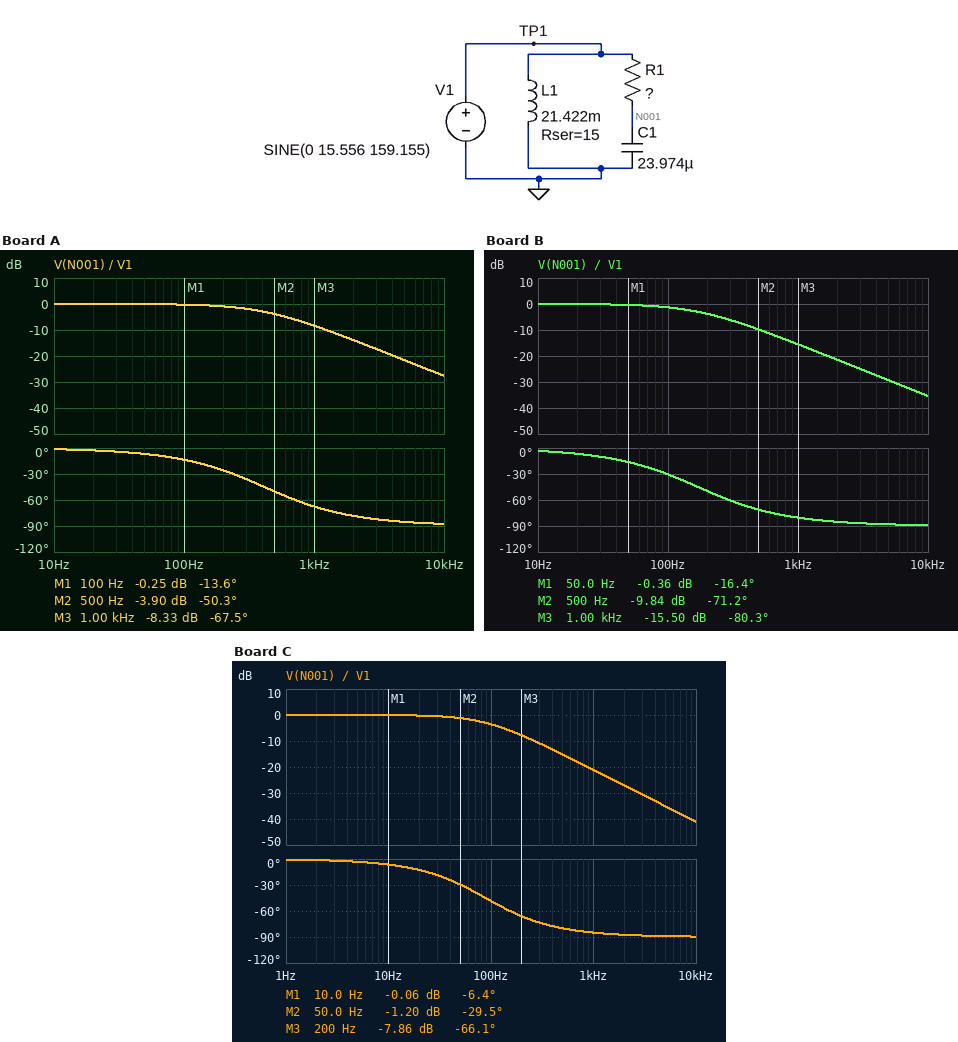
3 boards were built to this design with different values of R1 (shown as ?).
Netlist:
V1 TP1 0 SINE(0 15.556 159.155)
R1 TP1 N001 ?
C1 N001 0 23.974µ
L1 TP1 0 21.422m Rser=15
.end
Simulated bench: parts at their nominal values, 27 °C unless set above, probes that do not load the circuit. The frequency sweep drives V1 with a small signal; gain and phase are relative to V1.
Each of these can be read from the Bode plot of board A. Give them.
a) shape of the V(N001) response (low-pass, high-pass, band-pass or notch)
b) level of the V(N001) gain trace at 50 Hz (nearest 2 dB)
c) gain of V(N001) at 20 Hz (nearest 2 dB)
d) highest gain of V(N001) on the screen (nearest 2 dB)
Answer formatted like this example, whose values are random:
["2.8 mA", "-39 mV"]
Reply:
["low-pass", "0 dB", "0 dB", "0 dB"]
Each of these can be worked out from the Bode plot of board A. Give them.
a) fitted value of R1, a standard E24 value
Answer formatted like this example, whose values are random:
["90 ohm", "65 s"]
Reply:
["16 Ω"]
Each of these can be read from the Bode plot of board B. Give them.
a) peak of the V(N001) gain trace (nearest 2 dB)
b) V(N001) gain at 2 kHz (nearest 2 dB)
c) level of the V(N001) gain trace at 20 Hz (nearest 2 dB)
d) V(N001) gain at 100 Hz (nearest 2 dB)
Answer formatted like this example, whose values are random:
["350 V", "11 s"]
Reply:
["0 dB", "-22 dB", "0 dB", "-2 dB"]
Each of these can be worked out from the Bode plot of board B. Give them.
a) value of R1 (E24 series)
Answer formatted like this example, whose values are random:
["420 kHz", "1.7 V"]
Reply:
["39 Ω"]
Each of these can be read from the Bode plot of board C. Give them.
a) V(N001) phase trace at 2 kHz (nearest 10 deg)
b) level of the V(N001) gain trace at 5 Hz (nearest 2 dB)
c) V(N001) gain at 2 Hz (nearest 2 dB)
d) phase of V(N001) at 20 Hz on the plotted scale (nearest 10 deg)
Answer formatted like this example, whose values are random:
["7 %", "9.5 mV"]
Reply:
["-90 deg", "0 dB", "0 dB", "-10 deg"]
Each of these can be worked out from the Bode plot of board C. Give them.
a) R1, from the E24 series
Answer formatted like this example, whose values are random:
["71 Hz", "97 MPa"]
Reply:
["75 Ω"]
